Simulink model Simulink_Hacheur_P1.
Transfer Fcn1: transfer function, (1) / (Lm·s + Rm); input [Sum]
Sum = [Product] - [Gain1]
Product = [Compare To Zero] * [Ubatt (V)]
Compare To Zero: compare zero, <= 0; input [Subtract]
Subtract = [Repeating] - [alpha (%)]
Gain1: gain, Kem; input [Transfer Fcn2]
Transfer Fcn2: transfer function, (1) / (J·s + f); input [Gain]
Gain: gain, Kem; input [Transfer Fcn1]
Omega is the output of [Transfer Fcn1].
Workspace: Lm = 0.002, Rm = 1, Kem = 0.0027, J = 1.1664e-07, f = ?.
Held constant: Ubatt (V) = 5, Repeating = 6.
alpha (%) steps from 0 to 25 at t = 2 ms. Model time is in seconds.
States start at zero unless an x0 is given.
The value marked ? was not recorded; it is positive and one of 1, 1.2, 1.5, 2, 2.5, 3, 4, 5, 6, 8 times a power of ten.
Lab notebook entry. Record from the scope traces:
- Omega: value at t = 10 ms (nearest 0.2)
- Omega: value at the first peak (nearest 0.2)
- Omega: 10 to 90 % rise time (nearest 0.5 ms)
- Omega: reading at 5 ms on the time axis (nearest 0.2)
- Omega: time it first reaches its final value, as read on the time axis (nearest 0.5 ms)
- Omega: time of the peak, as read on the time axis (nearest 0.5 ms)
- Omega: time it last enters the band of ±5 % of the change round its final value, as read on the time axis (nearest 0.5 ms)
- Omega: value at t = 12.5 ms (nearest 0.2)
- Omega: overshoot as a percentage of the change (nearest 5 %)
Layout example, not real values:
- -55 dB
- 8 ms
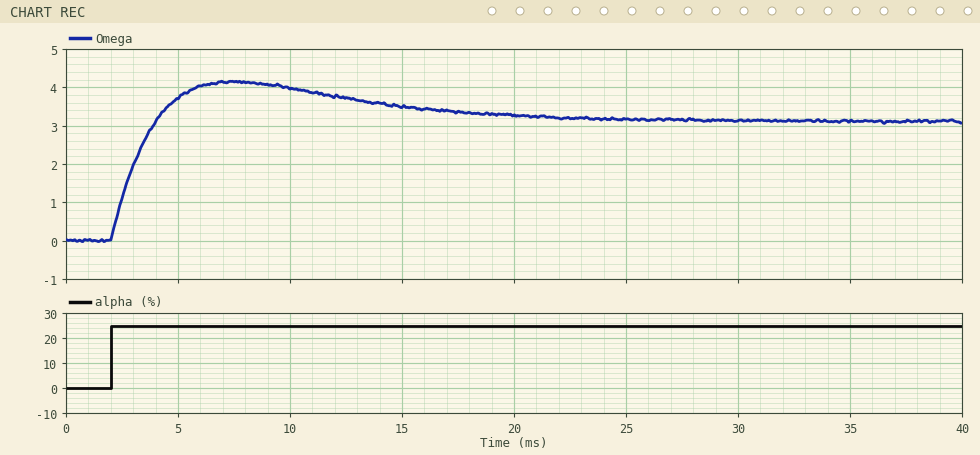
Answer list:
- 4.0
- 4.2
- 1.5 ms
- 3.8
- 4.0 ms
- 7.5 ms
- 20.0 ms
- 3.8
- 35 %
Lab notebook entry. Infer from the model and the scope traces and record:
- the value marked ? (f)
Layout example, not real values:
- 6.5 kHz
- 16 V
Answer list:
- 1.2e-05
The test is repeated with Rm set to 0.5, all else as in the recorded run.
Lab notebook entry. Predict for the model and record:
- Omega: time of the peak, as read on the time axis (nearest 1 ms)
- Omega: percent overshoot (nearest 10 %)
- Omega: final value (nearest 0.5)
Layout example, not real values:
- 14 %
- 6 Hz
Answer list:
- 9 ms
- 50 %
- 4.5
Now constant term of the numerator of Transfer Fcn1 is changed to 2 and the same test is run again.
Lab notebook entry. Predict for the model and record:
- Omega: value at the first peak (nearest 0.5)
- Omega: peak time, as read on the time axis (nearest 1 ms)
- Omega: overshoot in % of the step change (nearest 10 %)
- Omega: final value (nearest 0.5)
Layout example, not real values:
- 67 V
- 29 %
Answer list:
- 7.5
- 6 ms
- 70 %
- 4.5
